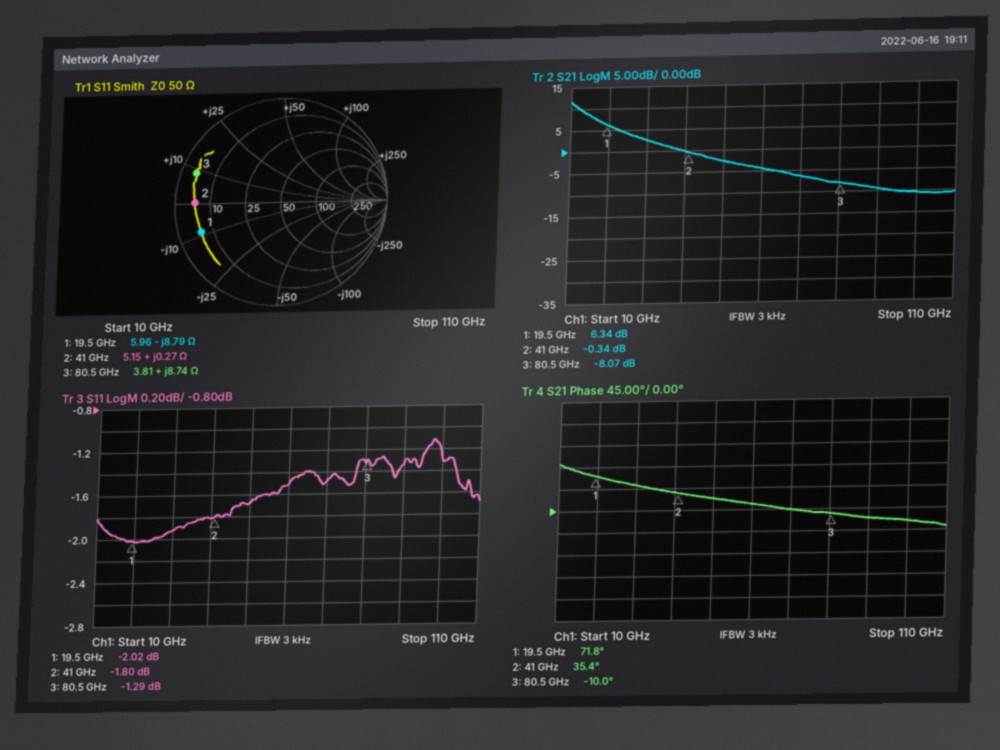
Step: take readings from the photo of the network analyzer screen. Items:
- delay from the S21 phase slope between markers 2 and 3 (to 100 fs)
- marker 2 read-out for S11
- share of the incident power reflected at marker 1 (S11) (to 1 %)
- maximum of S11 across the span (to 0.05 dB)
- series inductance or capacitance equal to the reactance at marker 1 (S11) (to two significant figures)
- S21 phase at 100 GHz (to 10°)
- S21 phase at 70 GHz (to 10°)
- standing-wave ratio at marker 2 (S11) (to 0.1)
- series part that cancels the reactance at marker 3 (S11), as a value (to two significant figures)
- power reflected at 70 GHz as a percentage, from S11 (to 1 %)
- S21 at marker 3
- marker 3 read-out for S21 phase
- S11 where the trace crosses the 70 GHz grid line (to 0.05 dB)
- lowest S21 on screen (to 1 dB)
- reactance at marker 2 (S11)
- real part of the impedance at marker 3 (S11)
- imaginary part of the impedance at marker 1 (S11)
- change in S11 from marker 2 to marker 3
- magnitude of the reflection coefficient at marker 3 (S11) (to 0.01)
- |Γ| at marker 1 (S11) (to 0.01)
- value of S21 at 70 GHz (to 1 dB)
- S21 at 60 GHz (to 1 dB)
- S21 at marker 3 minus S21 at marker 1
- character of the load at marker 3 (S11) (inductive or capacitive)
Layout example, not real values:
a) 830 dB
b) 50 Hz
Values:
a) 3.2 ps
b) -1.80 dB
c) 63 %
d) -1.10 dB
e) 930 fF
f) -30°
g) 0°
h) 9.7
i) 230 fF
j) 71 %
k) -8.07 dB
l) -10.0°
m) -1.50 dB
n) -11 dB
o) +0.27 Ω
p) 3.81 Ω
q) -8.79 Ω
r) 0.51 dB
s) 0.86
t) 0.79
u) -6 dB
v) -4 dB
w) -14.41 dB
x) inductive
